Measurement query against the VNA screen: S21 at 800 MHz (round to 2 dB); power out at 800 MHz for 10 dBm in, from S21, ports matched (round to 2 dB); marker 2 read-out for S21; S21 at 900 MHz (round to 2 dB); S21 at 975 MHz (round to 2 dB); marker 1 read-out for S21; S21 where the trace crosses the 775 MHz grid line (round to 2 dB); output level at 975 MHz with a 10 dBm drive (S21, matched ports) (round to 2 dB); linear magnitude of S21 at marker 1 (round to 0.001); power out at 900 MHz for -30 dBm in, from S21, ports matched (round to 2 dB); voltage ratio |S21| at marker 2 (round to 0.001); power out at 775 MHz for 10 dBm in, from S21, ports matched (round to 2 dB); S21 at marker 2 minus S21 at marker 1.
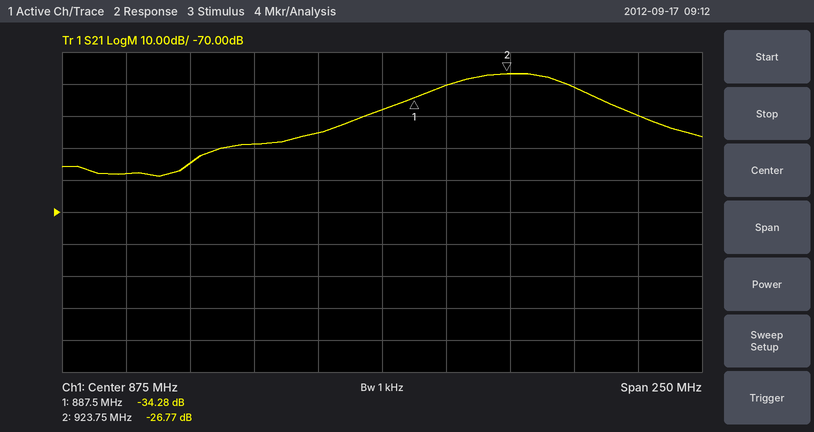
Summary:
-54 dB
-44 dBm
-26.77 dB
-30 dB
-40 dB
-34.28 dB
-58 dB
-30 dBm
0.019
-60 dBm
0.046
-48 dBm
7.51 dB
